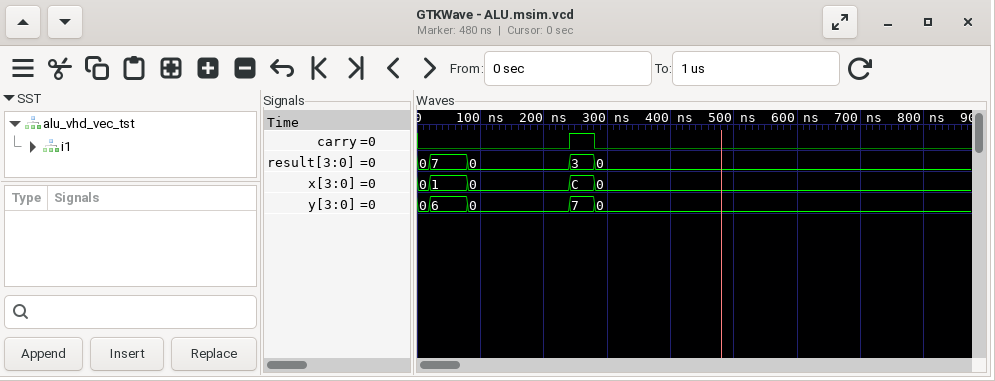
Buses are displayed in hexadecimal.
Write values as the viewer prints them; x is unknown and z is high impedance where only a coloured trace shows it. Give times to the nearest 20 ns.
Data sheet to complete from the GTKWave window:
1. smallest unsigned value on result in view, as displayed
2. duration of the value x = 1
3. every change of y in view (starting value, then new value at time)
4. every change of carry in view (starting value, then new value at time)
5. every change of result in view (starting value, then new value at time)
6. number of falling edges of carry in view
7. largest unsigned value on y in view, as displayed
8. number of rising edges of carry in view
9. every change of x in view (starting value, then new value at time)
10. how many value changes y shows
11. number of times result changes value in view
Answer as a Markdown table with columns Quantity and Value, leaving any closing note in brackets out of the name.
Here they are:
| Quantity | Value |
|---|---|
| smallest unsigned value on result in view, as displayed | 0 |
| duration of the value x = 1 | 60 ns |
| every change of y in view | 0, 6 at 20 ns, 0 at 80 ns, 7 at 240 ns, 0 at 280 ns |
| every change of carry in view | 0, 1 at 240 ns, 0 at 280 ns |
| every change of result in view | 0, 7 at 20 ns, 0 at 80 ns, 3 at 240 ns, 0 at 280 ns |
| number of falling edges of carry in view | 1 |
| largest unsigned value on y in view, as displayed | 7 |
| number of rising edges of carry in view | 1 |
| every change of x in view | 0, 1 at 20 ns, 0 at 80 ns, C at 240 ns, 0 at 280 ns |
| how many value changes y shows | 4 |
| number of times result changes value in view | 4 |
